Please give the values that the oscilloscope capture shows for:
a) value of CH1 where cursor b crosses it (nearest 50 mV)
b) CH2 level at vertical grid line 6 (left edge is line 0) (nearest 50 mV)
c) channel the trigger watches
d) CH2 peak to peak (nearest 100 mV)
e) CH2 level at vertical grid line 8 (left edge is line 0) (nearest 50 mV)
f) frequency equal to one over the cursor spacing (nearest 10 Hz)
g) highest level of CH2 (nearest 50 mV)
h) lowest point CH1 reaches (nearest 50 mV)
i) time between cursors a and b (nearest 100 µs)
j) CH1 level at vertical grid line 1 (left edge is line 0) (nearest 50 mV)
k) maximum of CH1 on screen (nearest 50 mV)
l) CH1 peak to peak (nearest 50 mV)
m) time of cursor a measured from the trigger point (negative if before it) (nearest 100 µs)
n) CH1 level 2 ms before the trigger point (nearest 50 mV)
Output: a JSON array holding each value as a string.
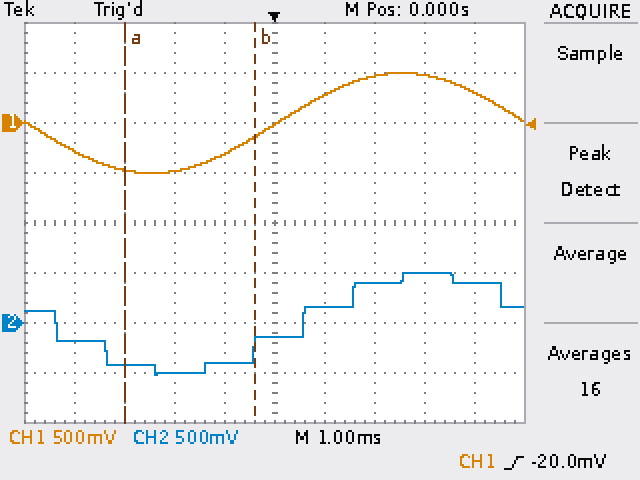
["-150 mV", "150 mV", "CH1", "1.00 V", "500 mV", "380 Hz", "500 mV", "-500 mV", "2.6 ms", "-300 mV", "500 mV", "1.00 V", "-3.0 ms", "-500 mV"]
